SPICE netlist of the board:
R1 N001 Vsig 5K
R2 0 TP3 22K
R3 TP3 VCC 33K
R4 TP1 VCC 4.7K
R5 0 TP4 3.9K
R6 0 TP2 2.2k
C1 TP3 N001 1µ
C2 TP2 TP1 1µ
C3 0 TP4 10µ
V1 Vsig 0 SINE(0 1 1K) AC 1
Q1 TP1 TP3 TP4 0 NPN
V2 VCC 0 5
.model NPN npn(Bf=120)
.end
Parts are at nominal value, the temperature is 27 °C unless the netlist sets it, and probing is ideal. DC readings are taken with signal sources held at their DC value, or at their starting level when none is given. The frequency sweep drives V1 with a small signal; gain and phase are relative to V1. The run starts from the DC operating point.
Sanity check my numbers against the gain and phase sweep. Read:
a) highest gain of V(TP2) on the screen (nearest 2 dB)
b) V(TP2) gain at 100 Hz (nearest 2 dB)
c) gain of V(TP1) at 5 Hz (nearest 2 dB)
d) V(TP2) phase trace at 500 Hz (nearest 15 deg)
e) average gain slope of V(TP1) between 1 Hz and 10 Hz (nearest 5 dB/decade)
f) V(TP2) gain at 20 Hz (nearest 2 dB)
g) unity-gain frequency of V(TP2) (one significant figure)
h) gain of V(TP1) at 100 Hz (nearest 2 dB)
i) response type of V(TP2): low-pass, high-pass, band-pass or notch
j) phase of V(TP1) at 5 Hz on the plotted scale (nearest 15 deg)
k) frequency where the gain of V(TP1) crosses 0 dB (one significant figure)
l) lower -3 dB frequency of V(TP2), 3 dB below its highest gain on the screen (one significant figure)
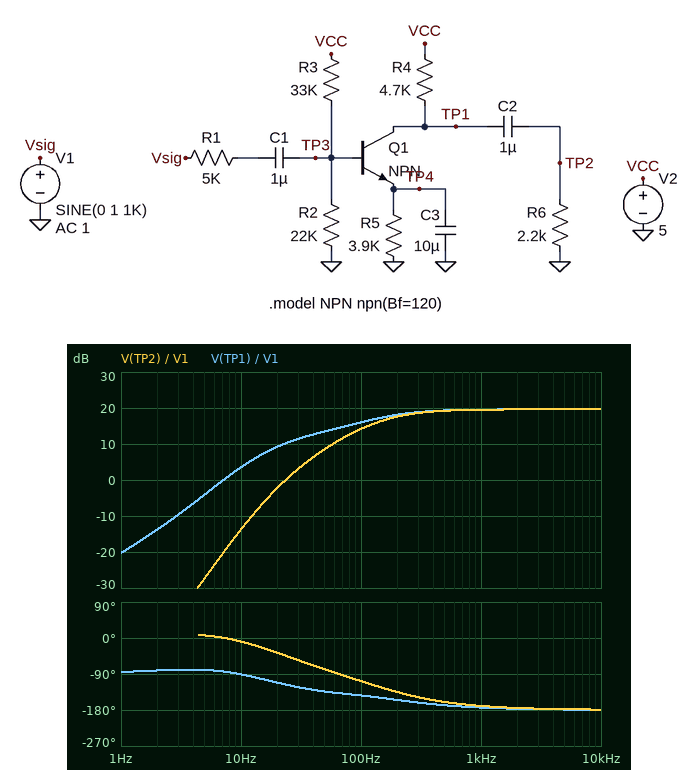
20 dB
14 dB
-4 dB
-165 deg
25 dB/decade
-2 dB
20 Hz
16 dB
high-pass
-75 deg
7 Hz
200 Hz
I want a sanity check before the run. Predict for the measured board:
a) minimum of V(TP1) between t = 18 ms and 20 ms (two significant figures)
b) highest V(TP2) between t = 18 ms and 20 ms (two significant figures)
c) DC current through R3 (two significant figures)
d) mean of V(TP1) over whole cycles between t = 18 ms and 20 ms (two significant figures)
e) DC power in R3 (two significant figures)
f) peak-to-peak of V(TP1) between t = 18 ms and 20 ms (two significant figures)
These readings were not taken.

1.6 V
670 mV
92 µA
3.0 V
280 µW
2.1 V
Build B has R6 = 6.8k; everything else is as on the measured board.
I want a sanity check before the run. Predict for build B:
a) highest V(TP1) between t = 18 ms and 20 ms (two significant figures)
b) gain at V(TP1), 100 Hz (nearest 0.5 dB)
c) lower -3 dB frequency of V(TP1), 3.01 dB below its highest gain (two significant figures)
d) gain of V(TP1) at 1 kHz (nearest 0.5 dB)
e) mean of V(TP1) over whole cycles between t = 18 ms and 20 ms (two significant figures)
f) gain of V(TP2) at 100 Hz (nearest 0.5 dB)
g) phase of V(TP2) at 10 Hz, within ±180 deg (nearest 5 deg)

4.3 V
20.0 dB
150 Hz
25.0 dB
3.3 V
19.5 dB
-20 deg
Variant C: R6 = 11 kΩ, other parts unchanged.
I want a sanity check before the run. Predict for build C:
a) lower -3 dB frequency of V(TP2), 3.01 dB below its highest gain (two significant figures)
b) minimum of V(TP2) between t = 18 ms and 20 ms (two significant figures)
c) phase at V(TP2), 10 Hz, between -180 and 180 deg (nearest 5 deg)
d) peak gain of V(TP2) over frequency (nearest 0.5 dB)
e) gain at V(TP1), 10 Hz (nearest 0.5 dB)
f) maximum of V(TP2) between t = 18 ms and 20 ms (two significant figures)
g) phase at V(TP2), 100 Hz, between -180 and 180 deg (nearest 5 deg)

150 Hz
-2.0 V
-30 deg
26.5 dB
3.0 dB
1.2 V
-115 deg
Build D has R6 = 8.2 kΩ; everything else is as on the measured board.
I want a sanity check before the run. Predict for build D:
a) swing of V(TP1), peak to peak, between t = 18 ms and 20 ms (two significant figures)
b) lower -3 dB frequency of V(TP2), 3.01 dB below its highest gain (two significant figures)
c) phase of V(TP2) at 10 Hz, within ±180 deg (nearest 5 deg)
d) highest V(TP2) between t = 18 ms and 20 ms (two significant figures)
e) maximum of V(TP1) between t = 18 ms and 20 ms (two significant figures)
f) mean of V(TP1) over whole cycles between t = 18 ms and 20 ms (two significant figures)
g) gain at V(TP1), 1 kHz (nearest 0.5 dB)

3.0 V
150 Hz
-25 deg
1.1 V
4.4 V
3.4 V
25.5 dB
